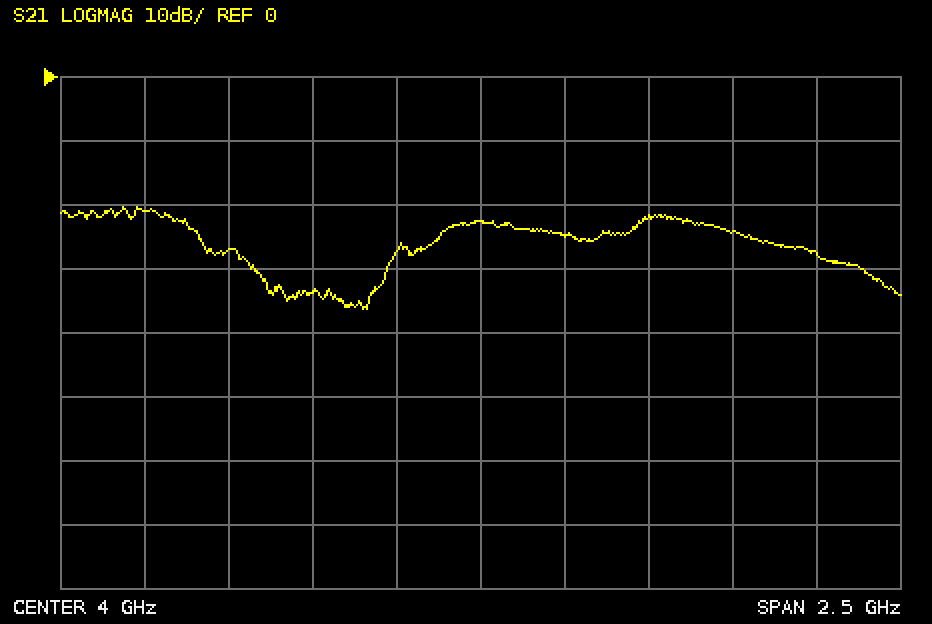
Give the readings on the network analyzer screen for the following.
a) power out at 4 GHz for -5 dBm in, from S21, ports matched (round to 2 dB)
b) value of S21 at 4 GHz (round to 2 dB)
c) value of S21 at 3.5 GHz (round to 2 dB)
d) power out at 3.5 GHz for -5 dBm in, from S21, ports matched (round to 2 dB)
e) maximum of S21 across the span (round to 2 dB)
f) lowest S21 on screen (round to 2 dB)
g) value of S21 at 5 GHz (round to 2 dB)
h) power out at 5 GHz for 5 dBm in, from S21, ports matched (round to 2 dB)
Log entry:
-28 dBm
-22 dB
-34 dB
-38 dBm
-20 dB
-36 dB
-28 dB
-22 dBm
